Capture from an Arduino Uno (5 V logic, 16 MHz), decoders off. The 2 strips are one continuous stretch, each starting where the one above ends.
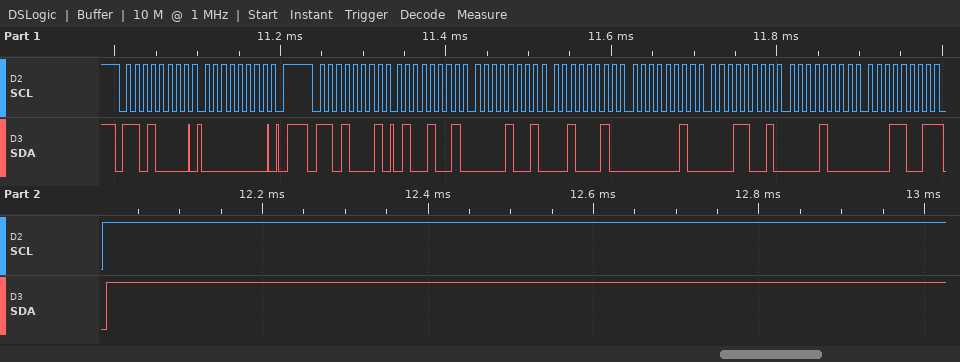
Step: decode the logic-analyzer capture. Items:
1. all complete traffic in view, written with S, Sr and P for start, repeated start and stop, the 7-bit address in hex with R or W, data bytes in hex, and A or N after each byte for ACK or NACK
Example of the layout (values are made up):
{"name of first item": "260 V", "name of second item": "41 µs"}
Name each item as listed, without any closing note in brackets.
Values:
{"all complete traffic in view, written with S, Sr and P for start, repeated start and stop, the 7-bit address in hex with R or W, data bytes in hex, and A or N after each byte for ACK or NACK": "S 68W A 00 A P S 68R A 49 A 09 A 22 A 02 A 19 A 08 A 19 N P"}
